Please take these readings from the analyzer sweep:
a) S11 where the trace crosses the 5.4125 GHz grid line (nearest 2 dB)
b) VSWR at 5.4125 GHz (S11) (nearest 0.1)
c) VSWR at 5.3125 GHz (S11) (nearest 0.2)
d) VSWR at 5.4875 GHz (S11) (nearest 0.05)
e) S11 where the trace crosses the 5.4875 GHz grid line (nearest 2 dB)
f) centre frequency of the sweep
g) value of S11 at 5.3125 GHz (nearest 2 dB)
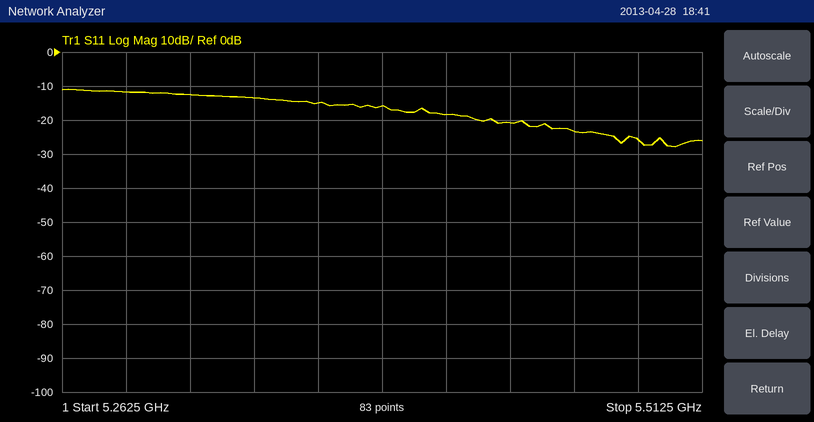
-18 dB
1.3
1.6
1.10
-26 dB
5.3875 GHz
-12 dB
